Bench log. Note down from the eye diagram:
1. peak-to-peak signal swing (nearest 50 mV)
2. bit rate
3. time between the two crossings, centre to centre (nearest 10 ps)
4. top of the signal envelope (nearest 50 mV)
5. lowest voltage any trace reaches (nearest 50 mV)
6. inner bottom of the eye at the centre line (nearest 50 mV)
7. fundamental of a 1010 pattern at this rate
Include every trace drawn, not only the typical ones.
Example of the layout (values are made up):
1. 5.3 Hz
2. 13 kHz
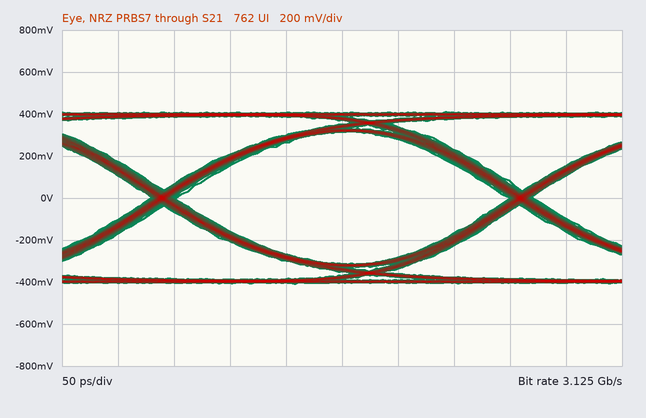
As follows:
1. 800 mV
2. 3.125 Gb/s
3. 320 ps
4. 400 mV
5. -400 mV
6. -300 mV
7. 1.5625 GHz
